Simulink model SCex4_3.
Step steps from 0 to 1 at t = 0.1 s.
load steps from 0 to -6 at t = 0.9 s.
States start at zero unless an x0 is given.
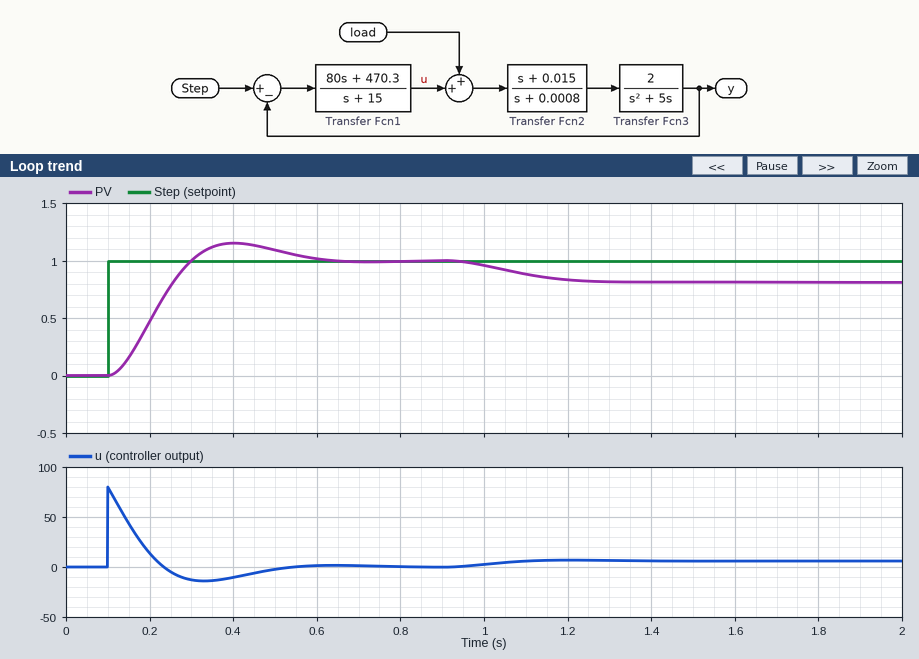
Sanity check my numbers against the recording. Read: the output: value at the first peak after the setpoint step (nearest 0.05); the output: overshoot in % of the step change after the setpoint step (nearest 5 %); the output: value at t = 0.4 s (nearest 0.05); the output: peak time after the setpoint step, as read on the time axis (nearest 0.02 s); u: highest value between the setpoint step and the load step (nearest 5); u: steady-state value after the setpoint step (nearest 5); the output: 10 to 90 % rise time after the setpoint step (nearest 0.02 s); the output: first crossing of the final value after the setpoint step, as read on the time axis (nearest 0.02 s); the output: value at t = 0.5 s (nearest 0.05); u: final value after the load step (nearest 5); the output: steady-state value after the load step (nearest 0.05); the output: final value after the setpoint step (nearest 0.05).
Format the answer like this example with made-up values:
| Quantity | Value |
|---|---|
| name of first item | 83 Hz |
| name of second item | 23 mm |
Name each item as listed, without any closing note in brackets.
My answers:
| Quantity | Value |
|---|---|
| the output: value at the first peak after the setpoint step | 1.15 |
| the output: overshoot in % of the step change after the setpoint step | 15 % |
| the output: value at t = 0.4 s | 1.15 |
| the output: peak time after the setpoint step, as read on the time axis | 0.40 s |
| u: highest value between the setpoint step and the load step | 80 |
| u: steady-state value after the setpoint step | 0 |
| the output: 10 to 90 % rise time after the setpoint step | 0.14 s |
| the output: first crossing of the final value after the setpoint step, as read on the time axis | 0.30 s |
| the output: value at t = 0.5 s | 1.10 |
| u: final value after the load step | 5 |
| the output: steady-state value after the load step | 0.80 |
| the output: final value after the setpoint step | 1.00 |
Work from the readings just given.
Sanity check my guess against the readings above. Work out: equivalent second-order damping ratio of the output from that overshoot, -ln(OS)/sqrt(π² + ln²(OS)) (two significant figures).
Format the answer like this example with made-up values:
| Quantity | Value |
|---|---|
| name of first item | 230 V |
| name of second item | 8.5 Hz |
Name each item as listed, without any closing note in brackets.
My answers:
| Quantity | Value |
|---|---|
| equivalent second-order damping ratio of the output from that overshoot, -ln(OS)/sqrt(π² + ln²(OS)) | 0.52 |
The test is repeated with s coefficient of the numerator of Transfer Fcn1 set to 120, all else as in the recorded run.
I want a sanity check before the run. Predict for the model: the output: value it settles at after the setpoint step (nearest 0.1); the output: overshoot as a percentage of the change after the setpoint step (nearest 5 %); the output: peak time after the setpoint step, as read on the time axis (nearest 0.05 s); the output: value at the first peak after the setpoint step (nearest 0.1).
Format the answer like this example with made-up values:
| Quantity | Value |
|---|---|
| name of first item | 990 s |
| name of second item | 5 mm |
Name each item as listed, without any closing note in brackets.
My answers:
| Quantity | Value |
|---|---|
| the output: value it settles at after the setpoint step | 1.0 |
| the output: overshoot as a percentage of the change after the setpoint step | 10 % |
| the output: peak time after the setpoint step, as read on the time axis | 0.35 s |
| the output: value at the first peak after the setpoint step | 1.1 |
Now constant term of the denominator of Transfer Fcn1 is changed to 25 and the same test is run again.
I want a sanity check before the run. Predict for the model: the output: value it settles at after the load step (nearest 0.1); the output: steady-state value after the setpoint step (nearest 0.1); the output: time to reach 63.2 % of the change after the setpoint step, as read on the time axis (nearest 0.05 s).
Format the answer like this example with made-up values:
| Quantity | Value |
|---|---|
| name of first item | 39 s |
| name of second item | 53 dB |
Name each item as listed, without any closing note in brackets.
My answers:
| Quantity | Value |
|---|---|
| the output: value it settles at after the load step | 0.7 |
| the output: steady-state value after the setpoint step | 1.0 |
| the output: time to reach 63.2 % of the change after the setpoint step, as read on the time axis | 0.25 s |
